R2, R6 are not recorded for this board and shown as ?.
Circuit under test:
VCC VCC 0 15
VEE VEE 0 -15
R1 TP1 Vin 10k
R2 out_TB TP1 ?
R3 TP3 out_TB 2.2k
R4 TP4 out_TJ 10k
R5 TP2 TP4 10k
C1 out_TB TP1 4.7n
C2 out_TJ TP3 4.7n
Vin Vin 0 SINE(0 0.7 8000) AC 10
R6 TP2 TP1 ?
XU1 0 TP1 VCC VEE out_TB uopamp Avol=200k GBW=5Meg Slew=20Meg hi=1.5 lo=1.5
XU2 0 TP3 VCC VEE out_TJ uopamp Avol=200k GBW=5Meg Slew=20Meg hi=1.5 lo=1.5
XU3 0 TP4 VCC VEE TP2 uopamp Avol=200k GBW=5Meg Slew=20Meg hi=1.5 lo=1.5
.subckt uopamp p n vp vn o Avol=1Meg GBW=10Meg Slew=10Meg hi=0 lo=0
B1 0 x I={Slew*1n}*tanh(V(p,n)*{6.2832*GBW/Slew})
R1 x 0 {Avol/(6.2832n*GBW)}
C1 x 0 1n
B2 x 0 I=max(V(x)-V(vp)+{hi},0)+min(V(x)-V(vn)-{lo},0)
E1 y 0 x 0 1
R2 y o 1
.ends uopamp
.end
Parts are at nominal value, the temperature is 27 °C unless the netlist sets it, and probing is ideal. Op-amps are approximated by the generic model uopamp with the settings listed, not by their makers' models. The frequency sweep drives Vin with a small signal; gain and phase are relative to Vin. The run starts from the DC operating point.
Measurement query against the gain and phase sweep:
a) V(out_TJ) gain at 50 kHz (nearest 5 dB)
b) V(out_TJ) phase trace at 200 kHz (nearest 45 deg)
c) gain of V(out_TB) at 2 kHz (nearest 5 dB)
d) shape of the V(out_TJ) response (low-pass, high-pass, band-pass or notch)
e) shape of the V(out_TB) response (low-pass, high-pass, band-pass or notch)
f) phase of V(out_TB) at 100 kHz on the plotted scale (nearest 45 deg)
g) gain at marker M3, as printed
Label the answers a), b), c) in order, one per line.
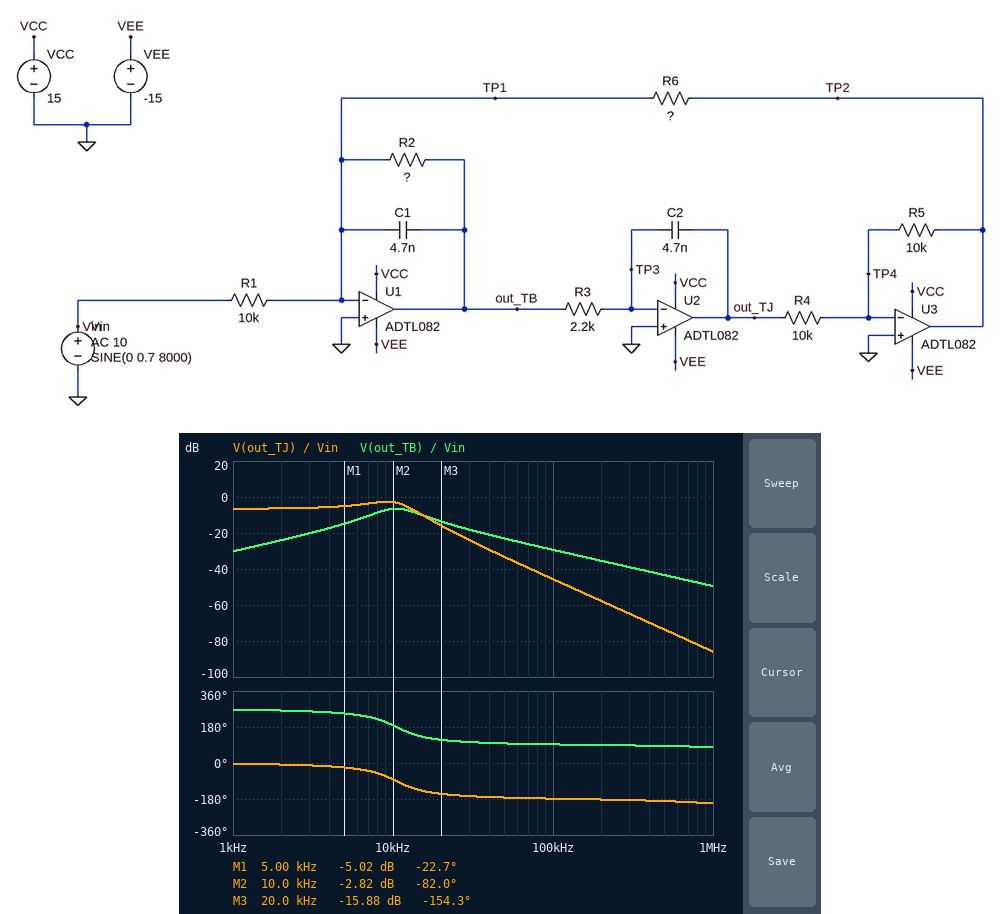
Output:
a) -35 dB
b) -180 deg
c) -25 dB
d) low-pass
e) band-pass
f) 90 deg
g) -15.88 dB
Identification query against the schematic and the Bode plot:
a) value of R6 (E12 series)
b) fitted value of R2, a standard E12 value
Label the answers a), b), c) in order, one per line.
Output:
a) 4.7 kΩ
b) 4.7 kΩ
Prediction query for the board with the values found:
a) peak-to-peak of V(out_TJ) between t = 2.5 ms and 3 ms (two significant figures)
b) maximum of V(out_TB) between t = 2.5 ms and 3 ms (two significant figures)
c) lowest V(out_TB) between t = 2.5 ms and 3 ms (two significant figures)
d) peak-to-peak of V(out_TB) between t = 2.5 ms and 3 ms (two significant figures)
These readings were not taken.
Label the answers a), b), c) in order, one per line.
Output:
a) 990 mV
b) 260 mV
c) -260 mV
d) 520 mV
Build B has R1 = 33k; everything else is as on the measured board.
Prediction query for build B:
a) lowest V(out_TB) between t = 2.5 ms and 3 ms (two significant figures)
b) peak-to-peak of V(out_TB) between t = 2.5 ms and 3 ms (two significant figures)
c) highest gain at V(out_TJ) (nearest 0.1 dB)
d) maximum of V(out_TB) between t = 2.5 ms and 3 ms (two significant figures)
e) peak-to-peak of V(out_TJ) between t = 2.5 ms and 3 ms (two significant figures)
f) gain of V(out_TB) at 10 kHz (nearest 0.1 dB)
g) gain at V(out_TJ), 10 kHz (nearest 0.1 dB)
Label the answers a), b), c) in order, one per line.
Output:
a) -78 mV
b) 160 mV
c) -13.0 dB
d) 78 mV
e) 300 mV
f) -16.9 dB
g) -13.2 dB
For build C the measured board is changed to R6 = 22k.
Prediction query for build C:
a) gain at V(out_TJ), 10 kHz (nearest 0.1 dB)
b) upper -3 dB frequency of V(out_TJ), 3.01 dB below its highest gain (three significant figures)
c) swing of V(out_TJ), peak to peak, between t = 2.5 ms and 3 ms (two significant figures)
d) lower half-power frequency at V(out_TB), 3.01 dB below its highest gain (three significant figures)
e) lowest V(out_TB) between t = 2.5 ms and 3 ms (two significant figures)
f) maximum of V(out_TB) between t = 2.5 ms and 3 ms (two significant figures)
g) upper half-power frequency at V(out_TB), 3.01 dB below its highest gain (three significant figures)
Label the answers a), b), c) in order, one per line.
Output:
a) -6.1 dB
b) 4.64 kHz
c) 1.0 V
d) 2.45 kHz
e) -270 mV
f) 270 mV
g) 9.63 kHz
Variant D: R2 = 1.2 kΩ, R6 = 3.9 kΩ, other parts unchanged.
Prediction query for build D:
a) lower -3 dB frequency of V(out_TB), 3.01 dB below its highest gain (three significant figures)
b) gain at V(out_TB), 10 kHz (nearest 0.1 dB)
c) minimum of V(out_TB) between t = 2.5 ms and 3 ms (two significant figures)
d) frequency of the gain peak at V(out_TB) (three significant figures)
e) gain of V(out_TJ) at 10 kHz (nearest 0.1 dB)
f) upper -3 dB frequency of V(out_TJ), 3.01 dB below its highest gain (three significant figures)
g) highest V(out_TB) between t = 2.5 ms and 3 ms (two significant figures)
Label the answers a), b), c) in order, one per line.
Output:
a) 4.13 kHz
b) -18.4 dB
c) -81 mV
d) 11.5 kHz
e) -14.7 dB
f) 5.65 kHz
g) 81 mV
